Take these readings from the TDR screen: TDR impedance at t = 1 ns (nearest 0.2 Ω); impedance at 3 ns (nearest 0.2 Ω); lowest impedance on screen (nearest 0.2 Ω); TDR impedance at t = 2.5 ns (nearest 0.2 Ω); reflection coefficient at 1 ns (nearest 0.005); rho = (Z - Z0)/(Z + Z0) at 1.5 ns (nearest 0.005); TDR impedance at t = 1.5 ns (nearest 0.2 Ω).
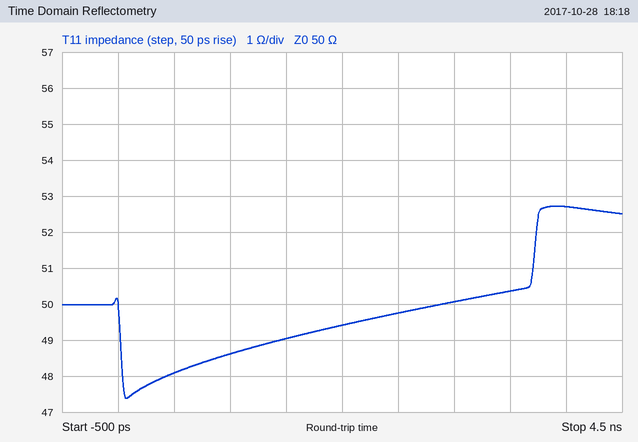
48.6 Ω
50.0 Ω
47.4 Ω
49.8 Ω
-0.015
-0.010
49.0 Ω
